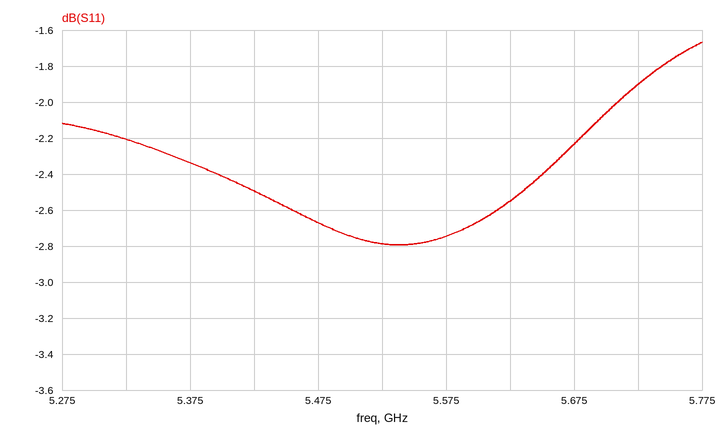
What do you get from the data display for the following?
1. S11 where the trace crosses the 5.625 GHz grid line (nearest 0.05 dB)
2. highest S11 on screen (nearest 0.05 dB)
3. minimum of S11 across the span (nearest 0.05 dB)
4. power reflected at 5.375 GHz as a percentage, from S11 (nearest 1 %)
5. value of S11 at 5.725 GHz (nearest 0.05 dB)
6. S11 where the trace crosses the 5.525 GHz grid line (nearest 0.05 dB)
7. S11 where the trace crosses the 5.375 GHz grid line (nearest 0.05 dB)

-2.55 dB
-1.65 dB
-2.80 dB
58 %
-1.90 dB
-2.80 dB
-2.35 dB
